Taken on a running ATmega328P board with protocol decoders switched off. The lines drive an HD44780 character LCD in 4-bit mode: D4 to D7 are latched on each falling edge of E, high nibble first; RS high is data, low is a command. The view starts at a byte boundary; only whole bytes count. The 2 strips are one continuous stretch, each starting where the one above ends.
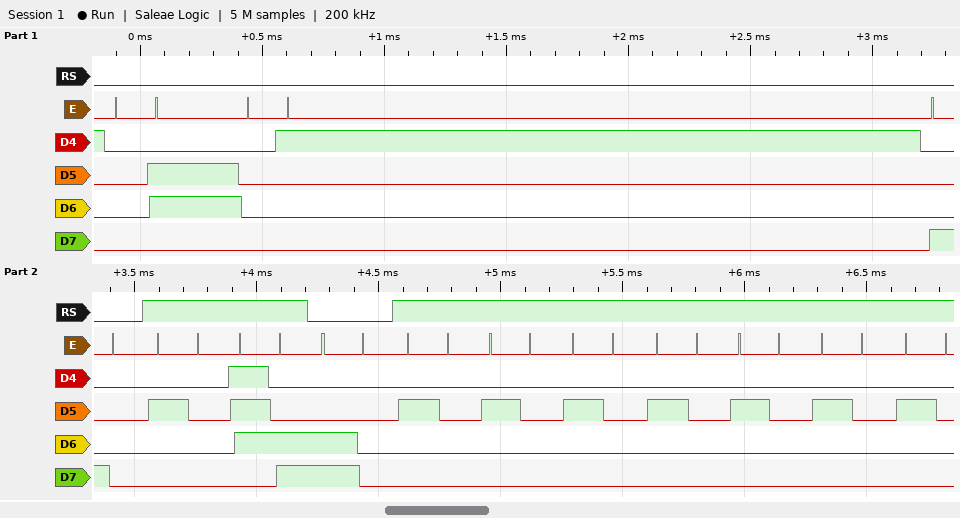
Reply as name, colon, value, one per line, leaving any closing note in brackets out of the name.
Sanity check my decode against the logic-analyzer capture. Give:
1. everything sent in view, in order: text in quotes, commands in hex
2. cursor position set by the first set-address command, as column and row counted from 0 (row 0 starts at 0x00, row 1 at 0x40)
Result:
everything sent in view, in order: text in quotes, commands in hex: 0x06 0x01 0x80 " |" 0xC0 "       "
cursor position set by the first set-address command, as column and row counted from 0: column 0, row 0
